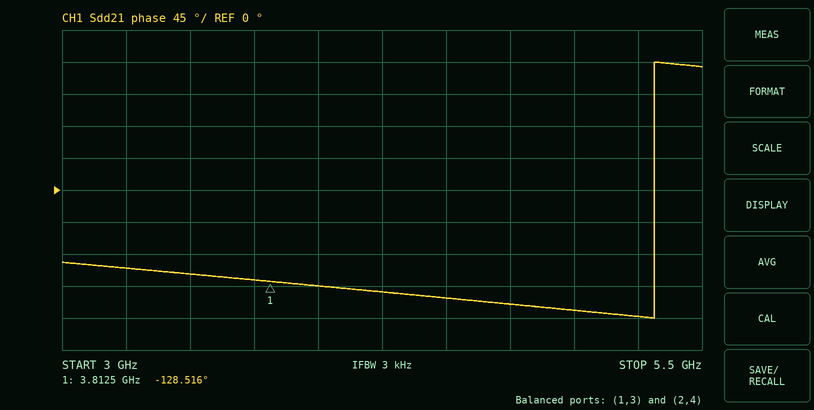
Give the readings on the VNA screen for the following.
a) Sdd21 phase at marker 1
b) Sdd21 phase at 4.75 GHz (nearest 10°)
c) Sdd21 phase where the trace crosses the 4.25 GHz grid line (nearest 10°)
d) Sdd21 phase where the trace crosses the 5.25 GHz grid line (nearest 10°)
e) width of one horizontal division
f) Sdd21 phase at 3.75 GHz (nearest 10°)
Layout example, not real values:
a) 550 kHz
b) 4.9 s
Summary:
a) -128.516°
b) -160°
c) -140°
d) -180°
e) 250 MHz
f) -130°
